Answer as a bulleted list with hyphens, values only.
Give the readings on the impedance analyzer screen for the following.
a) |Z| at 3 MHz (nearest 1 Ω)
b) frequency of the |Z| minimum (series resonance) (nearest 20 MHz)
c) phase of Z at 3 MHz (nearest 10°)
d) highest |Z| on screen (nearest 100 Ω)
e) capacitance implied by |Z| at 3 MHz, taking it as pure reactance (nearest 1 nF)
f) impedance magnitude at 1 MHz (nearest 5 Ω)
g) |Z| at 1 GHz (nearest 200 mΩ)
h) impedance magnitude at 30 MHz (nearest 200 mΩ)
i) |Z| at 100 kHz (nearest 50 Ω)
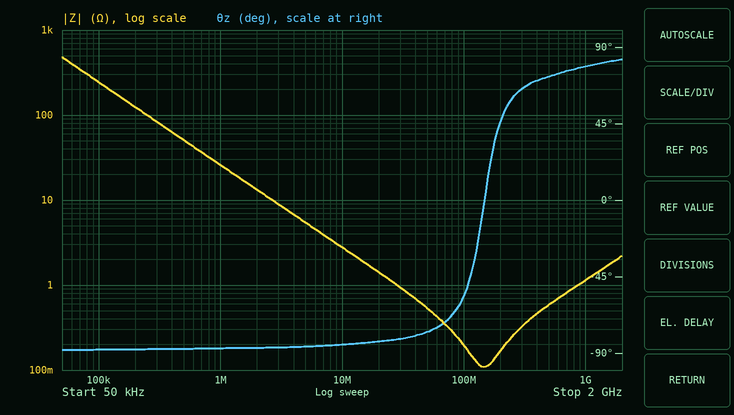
- 9 Ω
- 140 MHz
- -90°
- 500 Ω
- 6 nF
- 25 Ω
- 1.2 Ω
- 1.0 Ω
- 250 Ω
